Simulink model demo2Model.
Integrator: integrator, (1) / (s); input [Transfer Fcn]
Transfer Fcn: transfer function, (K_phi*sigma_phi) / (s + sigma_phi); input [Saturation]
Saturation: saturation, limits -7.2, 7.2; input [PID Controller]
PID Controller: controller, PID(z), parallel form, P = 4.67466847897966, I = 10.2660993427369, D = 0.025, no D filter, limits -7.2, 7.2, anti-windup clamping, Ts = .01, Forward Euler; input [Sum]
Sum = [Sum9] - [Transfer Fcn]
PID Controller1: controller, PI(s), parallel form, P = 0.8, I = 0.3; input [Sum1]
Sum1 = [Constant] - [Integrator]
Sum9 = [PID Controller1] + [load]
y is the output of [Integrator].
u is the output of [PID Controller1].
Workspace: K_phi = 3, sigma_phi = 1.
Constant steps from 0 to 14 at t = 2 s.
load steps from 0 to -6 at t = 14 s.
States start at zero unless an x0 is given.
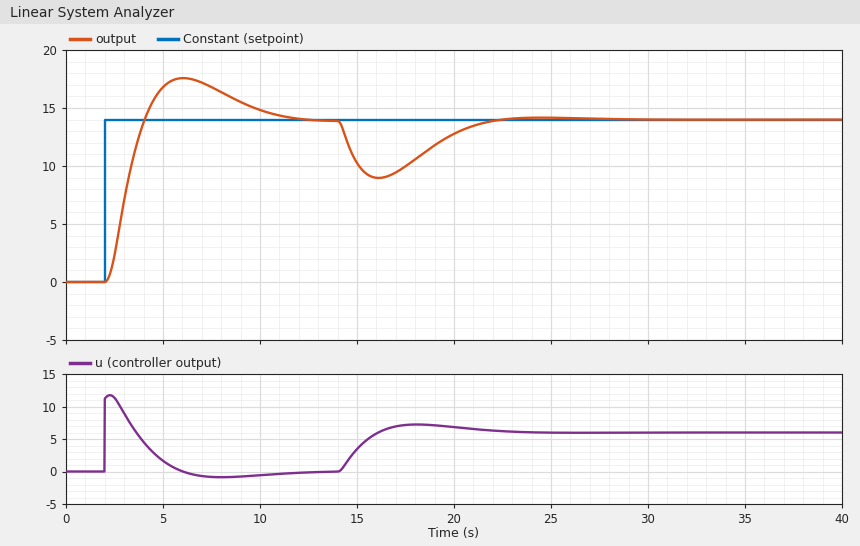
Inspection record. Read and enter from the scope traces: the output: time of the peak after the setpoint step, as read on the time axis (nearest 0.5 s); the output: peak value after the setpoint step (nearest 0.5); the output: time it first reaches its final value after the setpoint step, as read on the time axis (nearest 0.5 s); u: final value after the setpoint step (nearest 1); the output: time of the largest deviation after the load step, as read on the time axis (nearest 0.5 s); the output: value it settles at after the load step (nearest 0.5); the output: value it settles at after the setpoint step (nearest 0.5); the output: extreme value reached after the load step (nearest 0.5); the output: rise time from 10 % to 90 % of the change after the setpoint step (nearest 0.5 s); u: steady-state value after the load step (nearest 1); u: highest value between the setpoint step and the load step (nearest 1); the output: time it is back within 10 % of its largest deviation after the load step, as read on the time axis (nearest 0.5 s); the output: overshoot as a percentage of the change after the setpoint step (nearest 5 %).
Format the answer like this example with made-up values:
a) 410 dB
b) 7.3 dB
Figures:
a) 6.0 s
b) 17.5
c) 4.0 s
d) 0
e) 16.0 s
f) 14.0
g) 14.0
h) 9.0
i) 1.5 s
j) 6
k) 12
l) 21.0 s
m) 25 %
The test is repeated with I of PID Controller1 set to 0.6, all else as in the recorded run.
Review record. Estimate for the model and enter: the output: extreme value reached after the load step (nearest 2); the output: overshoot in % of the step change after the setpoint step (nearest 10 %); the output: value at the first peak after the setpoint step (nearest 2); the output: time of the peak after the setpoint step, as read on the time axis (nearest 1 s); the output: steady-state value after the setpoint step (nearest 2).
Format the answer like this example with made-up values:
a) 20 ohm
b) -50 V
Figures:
a) 10
b) 40 %
c) 20
d) 5 s
e) 14
